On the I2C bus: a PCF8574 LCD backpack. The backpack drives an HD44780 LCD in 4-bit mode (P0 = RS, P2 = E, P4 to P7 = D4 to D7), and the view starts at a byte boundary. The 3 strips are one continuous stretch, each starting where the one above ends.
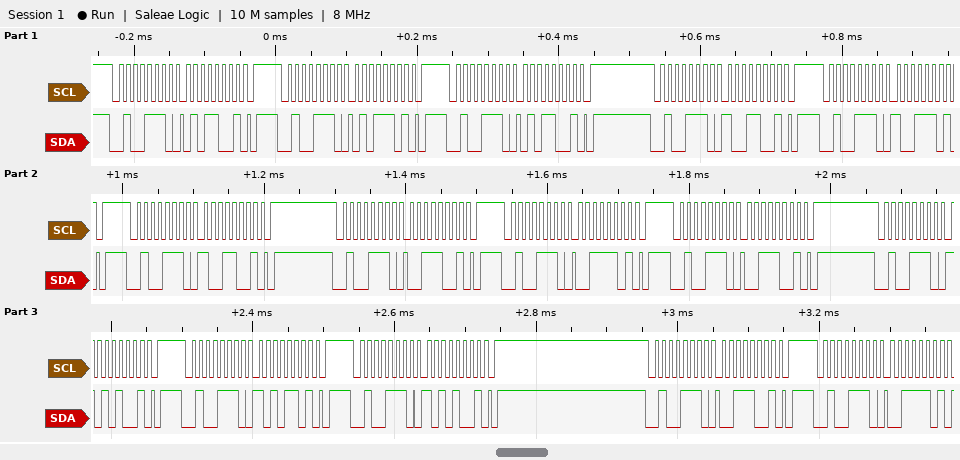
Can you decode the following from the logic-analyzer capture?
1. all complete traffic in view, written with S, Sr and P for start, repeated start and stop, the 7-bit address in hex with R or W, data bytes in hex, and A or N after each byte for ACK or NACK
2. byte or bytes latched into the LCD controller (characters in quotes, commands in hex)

S 27W A 59 A P S 27W A 5D A P S 27W A 59 A P S 27W A 99 A P S 27W A 9D A P S 27W A 99 A P S 27W A 39 A P S 27W A 3D A P S 27W A 39 A P S 27W A A9 A P S 27W A AD A P S 27W A A9 A P S 27W A 39 A P S 27W A 3D A
'Y' ':'
